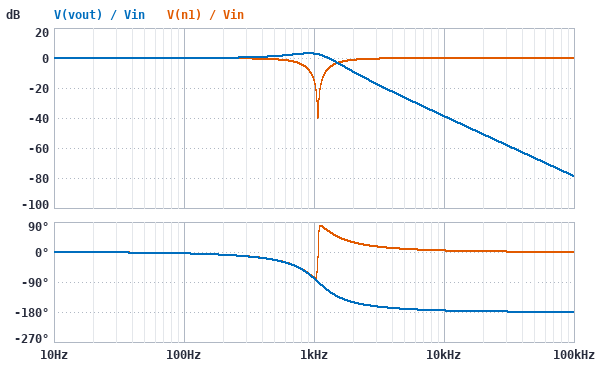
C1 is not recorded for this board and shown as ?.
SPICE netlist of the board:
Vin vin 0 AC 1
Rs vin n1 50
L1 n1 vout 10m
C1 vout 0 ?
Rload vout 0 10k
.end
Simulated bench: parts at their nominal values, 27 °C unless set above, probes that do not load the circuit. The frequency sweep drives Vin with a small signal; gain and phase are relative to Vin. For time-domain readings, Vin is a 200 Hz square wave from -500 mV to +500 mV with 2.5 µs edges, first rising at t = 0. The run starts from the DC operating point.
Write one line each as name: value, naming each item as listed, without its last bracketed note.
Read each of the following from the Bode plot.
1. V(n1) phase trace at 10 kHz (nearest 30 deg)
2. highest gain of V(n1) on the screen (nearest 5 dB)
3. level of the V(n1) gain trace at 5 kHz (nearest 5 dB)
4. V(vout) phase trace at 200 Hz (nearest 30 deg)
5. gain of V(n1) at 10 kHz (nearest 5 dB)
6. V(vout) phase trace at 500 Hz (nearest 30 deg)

V(n1) phase trace at 10 kHz: 0 deg
highest gain of V(n1) on the screen: 0 dB
level of the V(n1) gain trace at 5 kHz: 0 dB
V(vout) phase trace at 200 Hz: 0 deg
gain of V(n1) at 10 kHz: 0 dB
V(vout) phase trace at 500 Hz: -30 deg
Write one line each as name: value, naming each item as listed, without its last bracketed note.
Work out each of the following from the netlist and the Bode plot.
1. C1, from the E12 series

C1, from the E12 series: 2.2 µF
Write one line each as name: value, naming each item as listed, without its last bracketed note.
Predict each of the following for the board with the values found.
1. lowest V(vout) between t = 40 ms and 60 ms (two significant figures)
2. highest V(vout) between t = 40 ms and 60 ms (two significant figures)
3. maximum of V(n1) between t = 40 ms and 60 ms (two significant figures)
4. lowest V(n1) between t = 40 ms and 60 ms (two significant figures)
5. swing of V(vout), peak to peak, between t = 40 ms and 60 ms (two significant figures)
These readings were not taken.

lowest V(vout) between t = 40 ms and 60 ms: -780 mV
highest V(vout) between t = 40 ms and 60 ms: 780 mV
maximum of V(n1) between t = 40 ms and 60 ms: 630 mV
lowest V(n1) between t = 40 ms and 60 ms: -630 mV
swing of V(vout), peak to peak, between t = 40 ms and 60 ms: 1.6 V
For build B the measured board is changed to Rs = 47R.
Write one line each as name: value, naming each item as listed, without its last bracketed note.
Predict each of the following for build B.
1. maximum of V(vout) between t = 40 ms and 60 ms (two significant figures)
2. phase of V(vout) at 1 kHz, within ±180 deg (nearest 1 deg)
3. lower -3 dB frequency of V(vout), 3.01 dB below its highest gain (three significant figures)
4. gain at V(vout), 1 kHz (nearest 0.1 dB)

maximum of V(vout) between t = 40 ms and 60 ms: 810 mV
phase of V(vout) at 1 kHz, within ±180 deg: -78 deg
lower -3 dB frequency of V(vout), 3.01 dB below its highest gain: 333 Hz
gain at V(vout), 1 kHz: 3.5 dB
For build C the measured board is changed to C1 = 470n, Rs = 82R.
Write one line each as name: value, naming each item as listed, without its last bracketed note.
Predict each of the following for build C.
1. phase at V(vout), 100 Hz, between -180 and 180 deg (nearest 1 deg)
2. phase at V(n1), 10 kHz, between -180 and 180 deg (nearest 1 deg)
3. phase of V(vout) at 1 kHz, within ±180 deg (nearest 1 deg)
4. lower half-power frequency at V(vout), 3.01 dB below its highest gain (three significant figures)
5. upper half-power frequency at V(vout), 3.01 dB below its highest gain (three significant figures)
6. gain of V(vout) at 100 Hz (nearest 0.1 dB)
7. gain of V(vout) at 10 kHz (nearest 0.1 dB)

phase at V(vout), 100 Hz, between -180 and 180 deg: -1 deg
phase at V(n1), 10 kHz, between -180 and 180 deg: 8 deg
phase of V(vout) at 1 kHz, within ±180 deg: -17 deg
lower half-power frequency at V(vout), 3.01 dB below its highest gain: 1.24 kHz
upper half-power frequency at V(vout), 3.01 dB below its highest gain: 2.74 kHz
gain of V(vout) at 100 Hz: -0.1 dB
gain of V(vout) at 10 kHz: -25.0 dB
